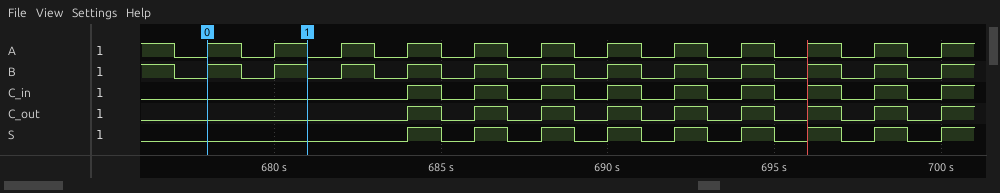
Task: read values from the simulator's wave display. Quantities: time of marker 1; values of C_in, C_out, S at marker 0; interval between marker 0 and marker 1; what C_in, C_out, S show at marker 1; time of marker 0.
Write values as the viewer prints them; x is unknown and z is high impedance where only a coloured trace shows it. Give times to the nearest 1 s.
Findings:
681 s
C_in=0, C_out=0, S=0
3 s
C_in=0, C_out=0, S=0
678 s
